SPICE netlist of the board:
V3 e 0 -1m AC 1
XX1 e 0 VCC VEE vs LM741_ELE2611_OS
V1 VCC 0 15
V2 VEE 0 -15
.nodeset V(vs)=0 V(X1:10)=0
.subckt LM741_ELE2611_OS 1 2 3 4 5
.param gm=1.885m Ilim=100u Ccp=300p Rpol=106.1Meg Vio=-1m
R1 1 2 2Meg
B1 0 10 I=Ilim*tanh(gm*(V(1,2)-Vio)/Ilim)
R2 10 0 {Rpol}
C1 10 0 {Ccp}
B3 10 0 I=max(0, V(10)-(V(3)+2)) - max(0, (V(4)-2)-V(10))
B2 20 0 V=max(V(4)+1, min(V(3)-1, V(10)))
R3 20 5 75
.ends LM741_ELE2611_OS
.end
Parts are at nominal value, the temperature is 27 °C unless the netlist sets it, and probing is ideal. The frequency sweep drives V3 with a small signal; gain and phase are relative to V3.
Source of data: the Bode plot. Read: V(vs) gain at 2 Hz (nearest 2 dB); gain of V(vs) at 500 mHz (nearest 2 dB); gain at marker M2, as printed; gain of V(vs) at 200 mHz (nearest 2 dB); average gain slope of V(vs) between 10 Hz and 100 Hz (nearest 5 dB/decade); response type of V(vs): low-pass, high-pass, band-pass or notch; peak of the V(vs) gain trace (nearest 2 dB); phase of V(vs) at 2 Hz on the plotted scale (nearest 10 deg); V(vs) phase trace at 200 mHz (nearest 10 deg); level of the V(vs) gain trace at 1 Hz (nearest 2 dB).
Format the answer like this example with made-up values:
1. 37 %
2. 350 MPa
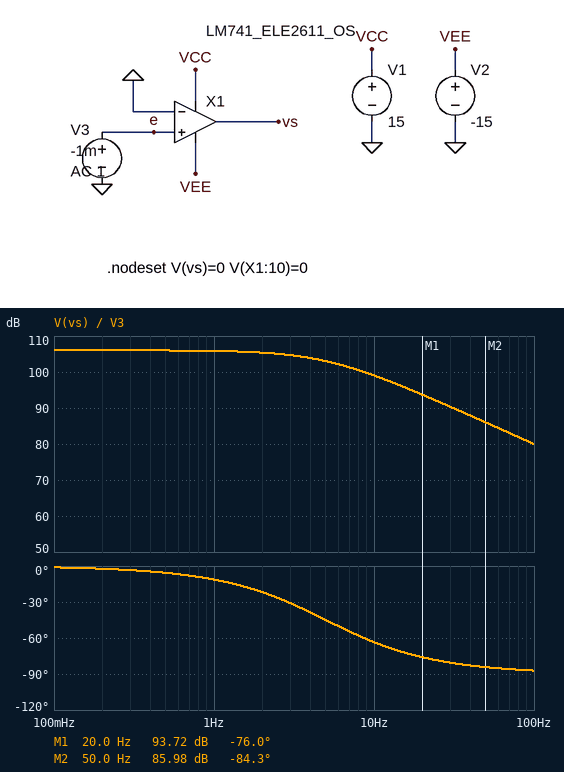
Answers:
1. 106 dB
2. 106 dB
3. 85.98 dB
4. 106 dB
5. -20 dB/decade
6. low-pass
7. 106 dB
8. -20 deg
9. 0 deg
10. 106 dB
